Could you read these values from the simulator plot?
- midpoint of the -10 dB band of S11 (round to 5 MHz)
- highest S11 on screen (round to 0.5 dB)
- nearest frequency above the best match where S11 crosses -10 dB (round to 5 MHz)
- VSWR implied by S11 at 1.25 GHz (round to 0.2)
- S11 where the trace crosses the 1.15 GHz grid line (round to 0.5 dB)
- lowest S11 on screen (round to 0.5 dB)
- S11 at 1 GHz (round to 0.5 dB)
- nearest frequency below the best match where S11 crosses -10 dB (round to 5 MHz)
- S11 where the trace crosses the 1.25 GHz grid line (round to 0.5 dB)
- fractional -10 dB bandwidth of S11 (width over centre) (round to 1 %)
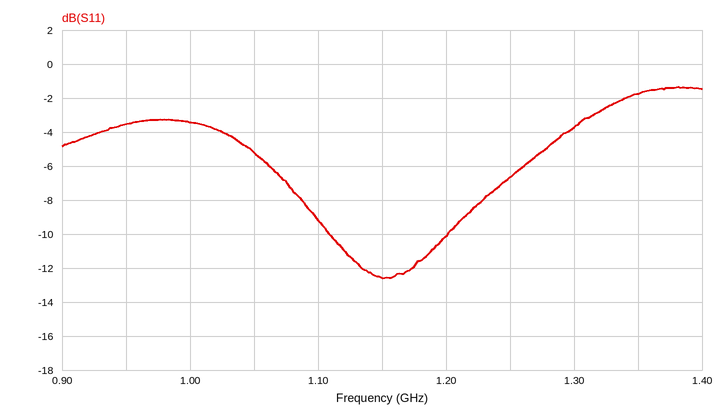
1.155 GHz
-1.5 dB
1.200 GHz
2.8
-12.5 dB
-12.5 dB
-3.5 dB
1.110 GHz
-6.5 dB
8 %
